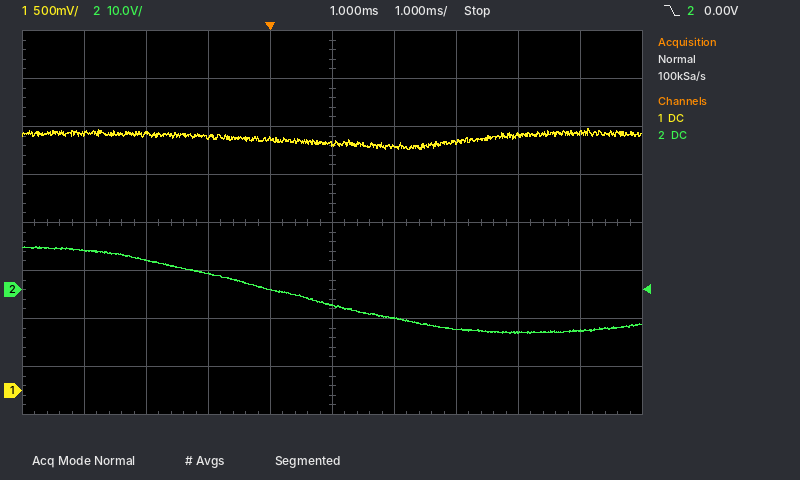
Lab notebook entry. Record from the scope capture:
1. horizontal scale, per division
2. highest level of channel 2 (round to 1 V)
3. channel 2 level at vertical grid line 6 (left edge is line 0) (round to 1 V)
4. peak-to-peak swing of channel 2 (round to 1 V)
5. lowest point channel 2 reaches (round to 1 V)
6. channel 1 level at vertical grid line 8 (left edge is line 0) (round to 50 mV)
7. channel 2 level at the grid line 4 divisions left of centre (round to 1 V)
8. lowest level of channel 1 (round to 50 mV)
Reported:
1 ms
9 V
-6 V
18 V
-9 V
2.65 V
8 V
2.50 V
